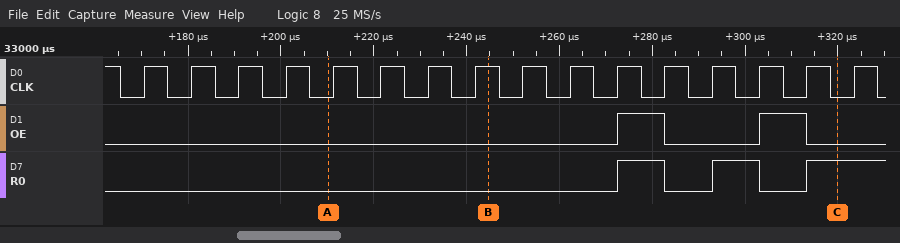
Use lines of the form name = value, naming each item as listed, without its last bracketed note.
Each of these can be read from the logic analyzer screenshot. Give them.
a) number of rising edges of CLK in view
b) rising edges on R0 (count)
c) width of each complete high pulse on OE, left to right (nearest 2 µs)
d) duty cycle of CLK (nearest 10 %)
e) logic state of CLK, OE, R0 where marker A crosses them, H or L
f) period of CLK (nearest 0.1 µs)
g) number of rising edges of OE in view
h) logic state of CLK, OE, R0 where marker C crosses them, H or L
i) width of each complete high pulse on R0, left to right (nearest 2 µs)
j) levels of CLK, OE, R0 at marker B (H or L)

number of rising edges of CLK in view = 16
rising edges on R0 = 3
width of each complete high pulse on OE, left to right = 10 µs, 10 µs
duty cycle of CLK = 50 %
logic state of CLK, OE, R0 where marker A crosses them, H or L = CLK=L, OE=L, R0=L
period of CLK = 10.2 µs
number of rising edges of OE in view = 2
logic state of CLK, OE, R0 where marker C crosses them, H or L = CLK=L, OE=L, R0=H
width of each complete high pulse on R0, left to right = 10 µs, 10 µs
levels of CLK, OE, R0 at marker B = CLK=H, OE=L, R0=L
